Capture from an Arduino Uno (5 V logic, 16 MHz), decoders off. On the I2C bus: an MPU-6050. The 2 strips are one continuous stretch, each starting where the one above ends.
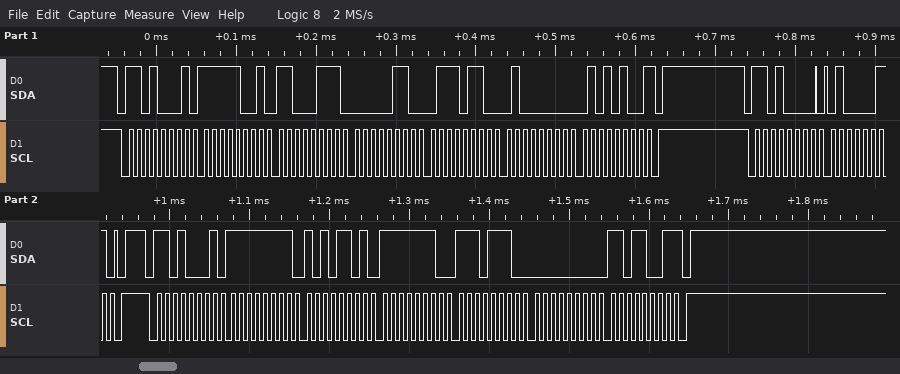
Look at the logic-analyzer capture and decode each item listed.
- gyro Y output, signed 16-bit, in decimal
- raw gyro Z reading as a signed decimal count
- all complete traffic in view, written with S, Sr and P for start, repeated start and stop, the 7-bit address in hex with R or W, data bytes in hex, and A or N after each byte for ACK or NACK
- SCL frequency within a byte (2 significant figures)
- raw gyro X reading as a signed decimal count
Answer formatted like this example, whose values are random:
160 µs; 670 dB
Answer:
-274; 217; S 68R A F9 A C7 A 06 A 76 A 40 A 54 N P S 68W A 43 A P S 68R A FF A AD A FE A EE A 00 A D9 N P; 100 kHz; -83
